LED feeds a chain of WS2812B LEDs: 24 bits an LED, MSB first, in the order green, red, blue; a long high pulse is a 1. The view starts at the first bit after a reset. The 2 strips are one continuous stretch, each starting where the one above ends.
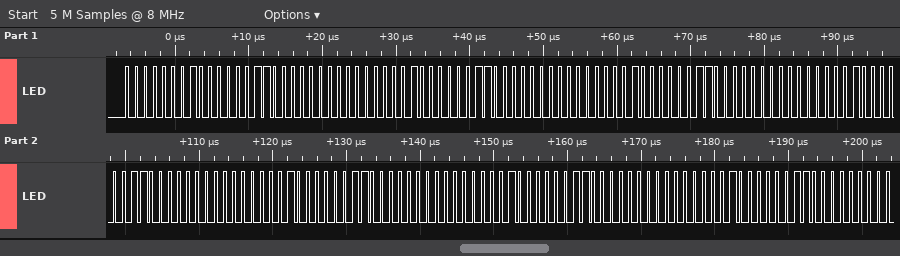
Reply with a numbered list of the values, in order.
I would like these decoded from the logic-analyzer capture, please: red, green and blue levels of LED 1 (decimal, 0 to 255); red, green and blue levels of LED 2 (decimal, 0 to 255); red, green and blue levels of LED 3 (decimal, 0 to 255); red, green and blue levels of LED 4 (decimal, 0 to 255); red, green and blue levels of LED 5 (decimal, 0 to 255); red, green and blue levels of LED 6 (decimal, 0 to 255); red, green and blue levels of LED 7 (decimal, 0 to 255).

1. 3, 1, 0
2. 3, 1, 0
3. 3, 1, 0
4. 3, 1, 0
5. 3, 1, 0
6. 3, 1, 0
7. 3, 1, 0
